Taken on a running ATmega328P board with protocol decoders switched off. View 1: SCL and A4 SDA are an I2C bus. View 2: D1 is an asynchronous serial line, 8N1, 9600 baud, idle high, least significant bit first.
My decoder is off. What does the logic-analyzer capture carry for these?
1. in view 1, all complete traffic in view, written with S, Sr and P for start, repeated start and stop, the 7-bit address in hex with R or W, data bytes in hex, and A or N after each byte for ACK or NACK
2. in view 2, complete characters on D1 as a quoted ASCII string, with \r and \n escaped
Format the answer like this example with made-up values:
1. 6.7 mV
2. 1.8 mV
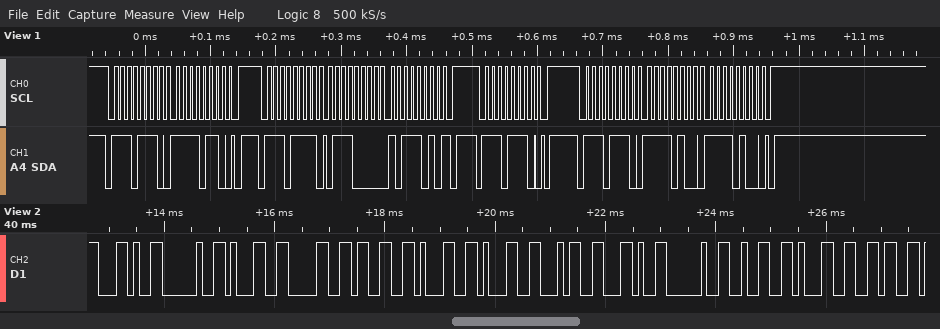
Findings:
1. S 77W A F6 A P S 77R A 70 A BA N P S 77W A P S 77W A F4 A F4 A P
2. ", 103114, 216"
